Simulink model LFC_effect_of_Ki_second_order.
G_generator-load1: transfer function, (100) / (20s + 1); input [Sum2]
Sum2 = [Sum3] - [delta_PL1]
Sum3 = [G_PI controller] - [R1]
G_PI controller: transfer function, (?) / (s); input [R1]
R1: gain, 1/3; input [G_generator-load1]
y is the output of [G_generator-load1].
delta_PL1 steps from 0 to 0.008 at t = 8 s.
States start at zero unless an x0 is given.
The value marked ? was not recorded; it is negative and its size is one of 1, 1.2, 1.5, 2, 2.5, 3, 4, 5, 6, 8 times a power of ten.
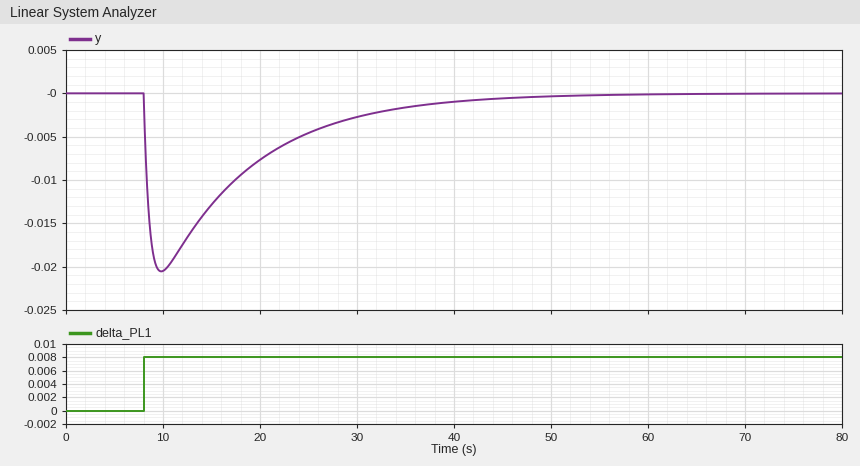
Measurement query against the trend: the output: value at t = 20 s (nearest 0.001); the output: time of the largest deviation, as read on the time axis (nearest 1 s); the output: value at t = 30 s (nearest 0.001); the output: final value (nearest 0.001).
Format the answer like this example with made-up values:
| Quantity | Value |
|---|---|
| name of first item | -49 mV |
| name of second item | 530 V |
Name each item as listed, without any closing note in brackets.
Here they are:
| Quantity | Value |
|---|---|
| the output: value at t = 20 s | -0.008 |
| the output: time of the largest deviation, as read on the time axis | 10 s |
| the output: value at t = 30 s | -0.003 |
| the output: final value | 0.000 |
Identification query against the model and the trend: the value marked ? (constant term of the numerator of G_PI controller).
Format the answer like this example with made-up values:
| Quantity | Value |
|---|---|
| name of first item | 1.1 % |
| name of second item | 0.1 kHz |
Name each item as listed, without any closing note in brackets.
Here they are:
| Quantity | Value |
|---|---|
| the value marked ? | -0.1 |
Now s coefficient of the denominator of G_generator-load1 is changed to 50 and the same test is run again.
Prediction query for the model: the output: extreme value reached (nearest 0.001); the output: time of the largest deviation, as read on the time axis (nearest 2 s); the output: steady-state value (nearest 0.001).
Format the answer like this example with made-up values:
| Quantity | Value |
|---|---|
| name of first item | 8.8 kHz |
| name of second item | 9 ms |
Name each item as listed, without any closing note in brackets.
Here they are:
| Quantity | Value |
|---|---|
| the output: extreme value reached | -0.019 |
| the output: time of the largest deviation, as read on the time axis | 12 s |
| the output: steady-state value | 0.000 |
